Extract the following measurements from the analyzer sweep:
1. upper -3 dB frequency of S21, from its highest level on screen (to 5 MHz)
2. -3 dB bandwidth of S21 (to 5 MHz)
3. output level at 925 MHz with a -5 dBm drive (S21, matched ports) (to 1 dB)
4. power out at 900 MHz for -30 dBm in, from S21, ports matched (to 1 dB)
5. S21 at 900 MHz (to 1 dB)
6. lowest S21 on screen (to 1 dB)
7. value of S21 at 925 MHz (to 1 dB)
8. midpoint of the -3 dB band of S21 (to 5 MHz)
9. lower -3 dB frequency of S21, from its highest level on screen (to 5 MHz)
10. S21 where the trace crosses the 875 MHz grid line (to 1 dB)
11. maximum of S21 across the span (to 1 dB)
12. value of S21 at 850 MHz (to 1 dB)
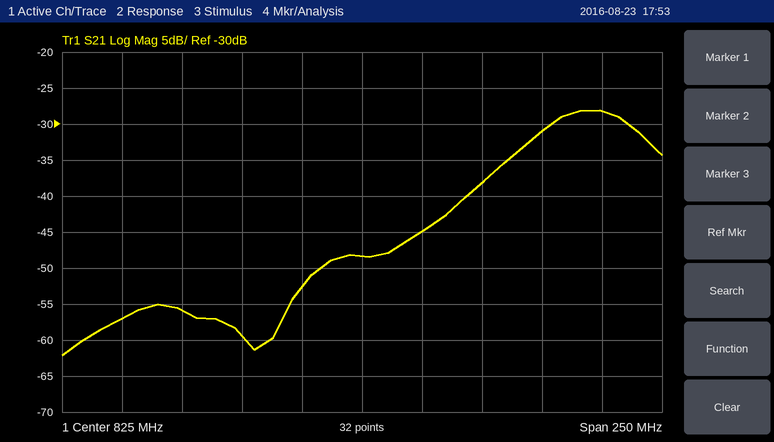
940 MHz
40 MHz
-33 dBm
-61 dBm
-31 dB
-62 dB
-28 dB
920 MHz
900 MHz
-38 dB
-28 dB
-45 dB
